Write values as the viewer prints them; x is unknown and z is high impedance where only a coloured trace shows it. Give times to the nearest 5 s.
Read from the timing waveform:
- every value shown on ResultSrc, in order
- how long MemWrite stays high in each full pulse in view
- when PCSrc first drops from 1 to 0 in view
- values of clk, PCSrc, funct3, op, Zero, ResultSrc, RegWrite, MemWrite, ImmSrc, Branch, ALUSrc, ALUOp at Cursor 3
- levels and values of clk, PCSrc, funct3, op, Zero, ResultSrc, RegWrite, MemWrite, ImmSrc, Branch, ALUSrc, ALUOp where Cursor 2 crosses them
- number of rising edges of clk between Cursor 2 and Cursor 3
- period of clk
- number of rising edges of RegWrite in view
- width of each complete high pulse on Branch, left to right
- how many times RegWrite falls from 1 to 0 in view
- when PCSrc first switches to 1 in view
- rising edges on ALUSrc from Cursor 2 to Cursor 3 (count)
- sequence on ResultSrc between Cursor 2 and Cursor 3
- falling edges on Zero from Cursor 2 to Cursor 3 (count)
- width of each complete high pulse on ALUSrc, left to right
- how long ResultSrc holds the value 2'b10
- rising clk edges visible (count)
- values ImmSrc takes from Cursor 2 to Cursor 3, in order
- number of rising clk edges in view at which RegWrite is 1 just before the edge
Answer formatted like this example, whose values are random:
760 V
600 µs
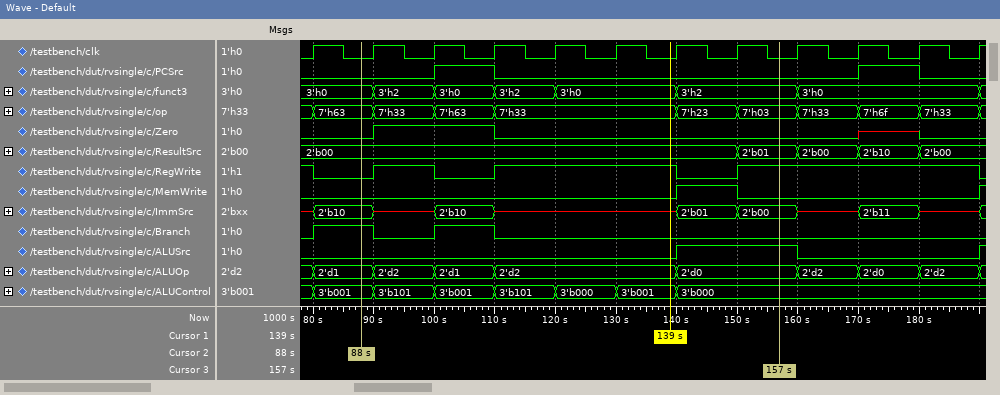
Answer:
2'b00, 2'b01, 2'b00, 2'b10, 2'b00
10 s
110 s
clk=0, PCSrc=0, funct3=3'h2, op=7'h03, Zero=0, ResultSrc=2'b01, RegWrite=1, MemWrite=0, ImmSrc=2'b00, Branch=0, ALUSrc=1, ALUOp=2'd0
clk=0, PCSrc=0, funct3=3'h0, op=7'h63, Zero=0, ResultSrc=2'b00, RegWrite=0, MemWrite=0, ImmSrc=2'b10, Branch=1, ALUSrc=0, ALUOp=2'd1
7
10 s
3
10 s, 10 s
4
100 s
1
2'b00, 2'b01
1
20 s
10 s
12
2'b10, x, 2'b10, x, 2'b01, 2'b00
9
